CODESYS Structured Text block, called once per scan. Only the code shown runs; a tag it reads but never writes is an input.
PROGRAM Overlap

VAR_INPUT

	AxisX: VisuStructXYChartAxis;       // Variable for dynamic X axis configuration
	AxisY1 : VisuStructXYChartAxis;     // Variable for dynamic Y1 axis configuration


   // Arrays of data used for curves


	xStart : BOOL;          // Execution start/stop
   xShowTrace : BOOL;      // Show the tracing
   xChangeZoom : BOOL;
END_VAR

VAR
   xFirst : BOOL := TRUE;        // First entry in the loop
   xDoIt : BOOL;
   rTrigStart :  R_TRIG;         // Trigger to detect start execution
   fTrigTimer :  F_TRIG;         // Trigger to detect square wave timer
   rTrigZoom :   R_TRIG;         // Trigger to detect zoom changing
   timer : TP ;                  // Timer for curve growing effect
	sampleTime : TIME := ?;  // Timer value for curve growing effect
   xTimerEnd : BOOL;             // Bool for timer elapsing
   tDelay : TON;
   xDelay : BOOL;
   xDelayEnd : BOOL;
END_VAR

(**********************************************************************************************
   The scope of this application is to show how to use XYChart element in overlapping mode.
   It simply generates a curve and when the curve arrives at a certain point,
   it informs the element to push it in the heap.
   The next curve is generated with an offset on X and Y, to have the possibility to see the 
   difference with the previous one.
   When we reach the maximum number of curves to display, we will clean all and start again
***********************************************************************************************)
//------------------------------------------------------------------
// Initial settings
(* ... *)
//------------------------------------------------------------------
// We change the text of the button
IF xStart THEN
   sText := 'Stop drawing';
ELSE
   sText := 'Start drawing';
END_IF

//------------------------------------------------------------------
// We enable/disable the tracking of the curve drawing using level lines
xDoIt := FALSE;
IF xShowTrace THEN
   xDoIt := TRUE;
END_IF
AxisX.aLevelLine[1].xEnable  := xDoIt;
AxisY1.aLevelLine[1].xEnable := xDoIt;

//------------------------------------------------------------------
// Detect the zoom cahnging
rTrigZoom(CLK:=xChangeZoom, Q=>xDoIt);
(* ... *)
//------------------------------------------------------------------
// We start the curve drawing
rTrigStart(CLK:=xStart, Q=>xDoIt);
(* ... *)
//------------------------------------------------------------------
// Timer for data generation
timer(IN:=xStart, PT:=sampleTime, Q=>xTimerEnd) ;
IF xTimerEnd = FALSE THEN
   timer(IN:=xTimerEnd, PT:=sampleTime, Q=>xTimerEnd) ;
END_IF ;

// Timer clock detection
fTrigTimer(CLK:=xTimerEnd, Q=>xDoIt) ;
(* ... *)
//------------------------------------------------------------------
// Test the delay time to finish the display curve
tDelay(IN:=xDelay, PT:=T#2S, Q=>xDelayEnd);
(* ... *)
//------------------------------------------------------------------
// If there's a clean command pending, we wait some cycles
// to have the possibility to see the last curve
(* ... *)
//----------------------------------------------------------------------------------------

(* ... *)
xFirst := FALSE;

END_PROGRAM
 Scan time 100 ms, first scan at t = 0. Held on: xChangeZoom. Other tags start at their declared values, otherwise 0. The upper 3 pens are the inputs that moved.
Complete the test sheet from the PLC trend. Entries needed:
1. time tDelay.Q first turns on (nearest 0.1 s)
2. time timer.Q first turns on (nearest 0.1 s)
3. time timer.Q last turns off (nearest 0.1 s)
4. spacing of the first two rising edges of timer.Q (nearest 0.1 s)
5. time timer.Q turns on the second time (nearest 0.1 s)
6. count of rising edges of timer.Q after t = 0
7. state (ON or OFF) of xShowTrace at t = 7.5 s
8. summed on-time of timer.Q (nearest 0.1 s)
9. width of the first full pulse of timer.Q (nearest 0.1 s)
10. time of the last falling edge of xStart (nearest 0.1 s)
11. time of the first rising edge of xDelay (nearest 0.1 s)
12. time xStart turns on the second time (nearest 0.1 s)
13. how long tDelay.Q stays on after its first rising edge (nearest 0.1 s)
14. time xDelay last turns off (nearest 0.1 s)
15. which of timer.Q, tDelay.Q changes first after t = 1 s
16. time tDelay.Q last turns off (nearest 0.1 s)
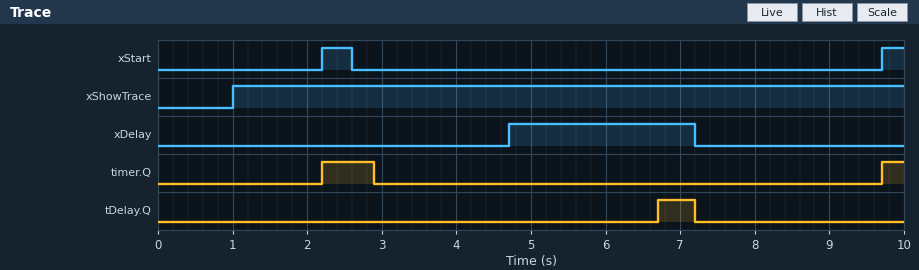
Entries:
6.7 s
2.2 s
2.9 s
7.5 s
9.7 s
2
ON
1.0 s
0.7 s
2.6 s
4.7 s
9.7 s
0.5 s
7.2 s
timer.Q
7.2 s
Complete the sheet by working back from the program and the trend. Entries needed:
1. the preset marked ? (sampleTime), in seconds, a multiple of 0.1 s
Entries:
0.7 s
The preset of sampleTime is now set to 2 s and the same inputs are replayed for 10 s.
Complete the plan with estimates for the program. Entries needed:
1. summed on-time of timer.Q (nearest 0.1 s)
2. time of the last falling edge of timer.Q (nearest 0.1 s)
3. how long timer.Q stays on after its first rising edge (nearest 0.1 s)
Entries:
2.3 s
4.2 s
2.0 s
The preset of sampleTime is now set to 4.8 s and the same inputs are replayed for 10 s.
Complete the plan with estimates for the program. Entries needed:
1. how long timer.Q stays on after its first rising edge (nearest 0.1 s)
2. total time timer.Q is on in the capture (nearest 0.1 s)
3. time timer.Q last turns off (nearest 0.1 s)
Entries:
4.8 s
5.1 s
7.0 s
